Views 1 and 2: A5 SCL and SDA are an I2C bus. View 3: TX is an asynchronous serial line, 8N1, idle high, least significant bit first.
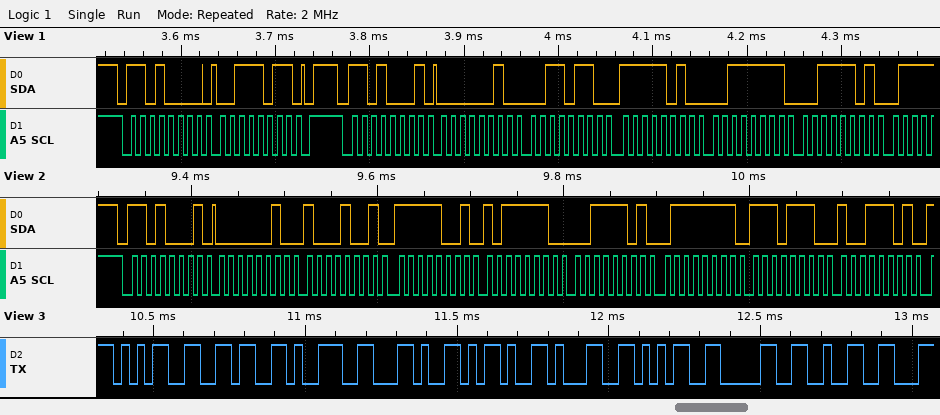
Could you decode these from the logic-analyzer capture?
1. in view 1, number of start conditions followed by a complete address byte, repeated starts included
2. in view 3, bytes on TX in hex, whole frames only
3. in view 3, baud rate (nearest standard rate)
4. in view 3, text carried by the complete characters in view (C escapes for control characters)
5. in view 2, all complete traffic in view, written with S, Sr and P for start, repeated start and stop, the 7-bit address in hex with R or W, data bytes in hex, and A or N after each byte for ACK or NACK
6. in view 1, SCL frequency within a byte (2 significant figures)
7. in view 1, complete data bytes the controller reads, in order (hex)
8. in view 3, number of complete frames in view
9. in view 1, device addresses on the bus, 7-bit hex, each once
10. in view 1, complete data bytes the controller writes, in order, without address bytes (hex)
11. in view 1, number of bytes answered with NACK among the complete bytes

2
35 36 39 2C 2D 31 35 30 32
38400 baud
"569,-1502"
S 68R A 02 A 89 A F9 A BE A 3D A 7F A EE A 9D A
100 kHz
02 36 FA 3F 3D
9
0x68
3B
0
